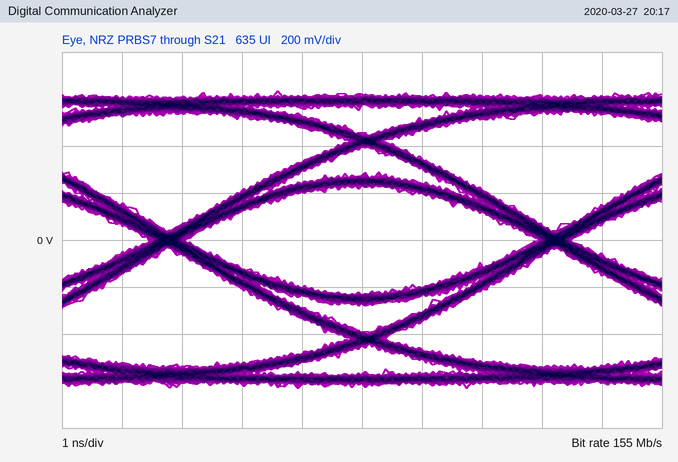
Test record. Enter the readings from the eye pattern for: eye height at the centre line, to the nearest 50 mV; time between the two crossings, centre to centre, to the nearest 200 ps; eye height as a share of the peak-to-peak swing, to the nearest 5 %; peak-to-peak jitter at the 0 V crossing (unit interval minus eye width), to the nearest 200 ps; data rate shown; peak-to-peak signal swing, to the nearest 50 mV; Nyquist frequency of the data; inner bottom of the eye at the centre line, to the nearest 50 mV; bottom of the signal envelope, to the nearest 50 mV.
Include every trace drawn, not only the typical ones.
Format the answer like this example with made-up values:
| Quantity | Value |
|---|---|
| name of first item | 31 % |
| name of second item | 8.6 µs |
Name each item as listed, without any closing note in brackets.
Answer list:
| Quantity | Value |
|---|---|
| eye height at the centre line, to the nearest 50 mV | 450 mV |
| time between the two crossings, centre to centre, to the nearest 200 ps | 6.4 ns |
| eye height as a share of the peak-to-peak swing, to the nearest 5 % | 35 % |
| peak-to-peak jitter at the 0 V crossing (unit interval minus eye width), to the nearest 200 ps | 600 ps |
| data rate shown | 155 Mb/s |
| peak-to-peak signal swing, to the nearest 50 mV | 1.25 V |
| Nyquist frequency of the data | 77.5 MHz |
| inner bottom of the eye at the centre line, to the nearest 50 mV | -250 mV |
| bottom of the signal envelope, to the nearest 50 mV | -650 mV |
